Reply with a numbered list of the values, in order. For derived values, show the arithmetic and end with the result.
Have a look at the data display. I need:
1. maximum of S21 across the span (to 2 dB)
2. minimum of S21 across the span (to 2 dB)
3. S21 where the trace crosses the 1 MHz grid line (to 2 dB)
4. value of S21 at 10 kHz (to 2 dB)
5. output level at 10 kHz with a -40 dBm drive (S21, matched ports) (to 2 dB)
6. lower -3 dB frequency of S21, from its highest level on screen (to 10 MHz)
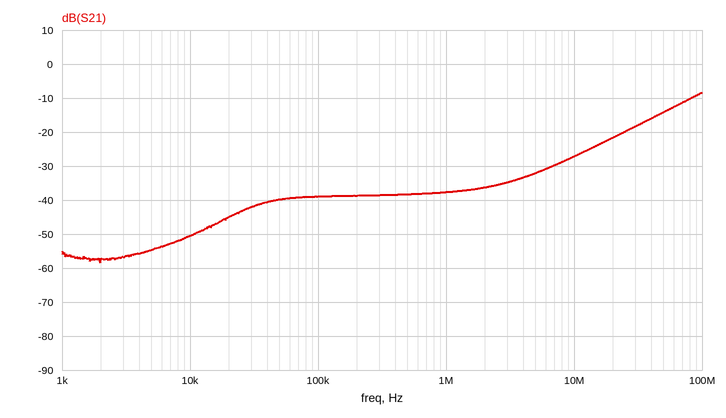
1. -8 dB
2. -58 dB
3. -38 dB
4. -50 dB
5. -40 dBm + (-50 dB) = -90 dBm
6. 70 MHz
